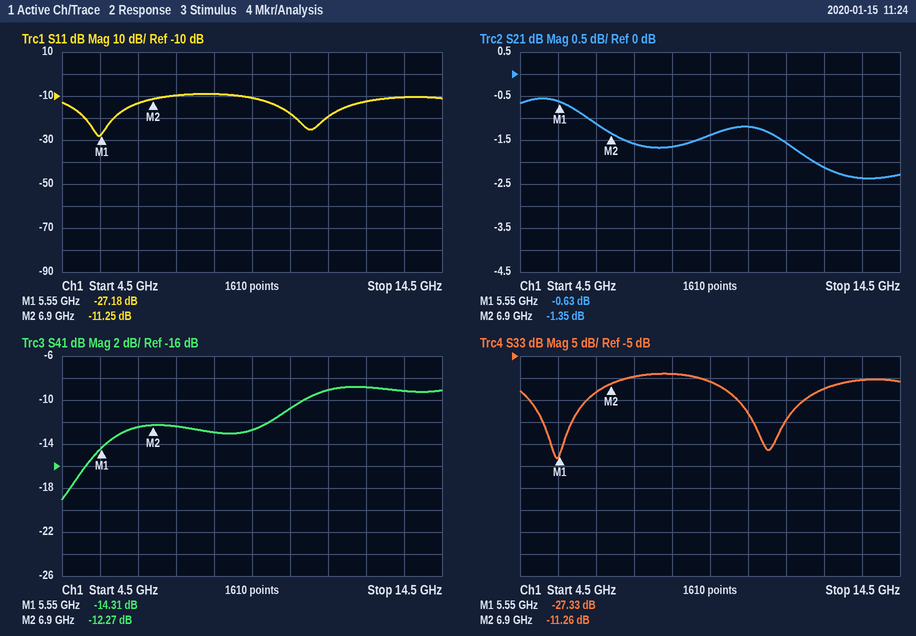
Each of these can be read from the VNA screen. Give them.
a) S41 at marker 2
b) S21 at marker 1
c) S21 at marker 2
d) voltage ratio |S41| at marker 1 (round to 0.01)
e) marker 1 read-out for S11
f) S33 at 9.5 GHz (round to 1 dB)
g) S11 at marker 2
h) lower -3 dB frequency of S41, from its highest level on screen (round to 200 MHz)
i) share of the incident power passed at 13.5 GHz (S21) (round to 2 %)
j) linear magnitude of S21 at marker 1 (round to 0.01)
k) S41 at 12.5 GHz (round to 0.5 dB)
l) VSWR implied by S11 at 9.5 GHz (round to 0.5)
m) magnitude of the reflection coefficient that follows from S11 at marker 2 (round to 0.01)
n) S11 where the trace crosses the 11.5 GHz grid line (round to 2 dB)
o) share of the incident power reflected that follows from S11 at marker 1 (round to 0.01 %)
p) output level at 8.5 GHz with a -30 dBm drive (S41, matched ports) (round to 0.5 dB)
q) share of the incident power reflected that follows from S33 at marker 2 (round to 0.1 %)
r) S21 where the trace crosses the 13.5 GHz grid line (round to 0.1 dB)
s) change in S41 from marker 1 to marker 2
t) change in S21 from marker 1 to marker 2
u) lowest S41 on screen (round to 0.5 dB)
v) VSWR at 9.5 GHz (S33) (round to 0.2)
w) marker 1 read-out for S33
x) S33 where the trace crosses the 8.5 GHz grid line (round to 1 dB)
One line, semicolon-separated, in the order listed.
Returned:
-12.27 dB; -0.63 dB; -1.35 dB; 0.19; -27.18 dB; -11 dB; -11.25 dB; 10.0 GHz; 58 %; 0.93; -9.0 dB; 2.0; 0.27; -20 dB; 0.19 %; -43.0 dBm; 7.5 %; -2.4 dB; 2.04 dB; -0.72 dB; -19.0 dB; 1.8; -27.33 dB; -9 dB
